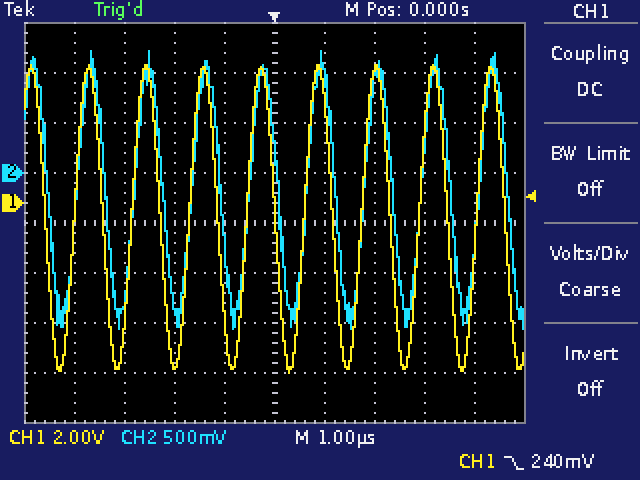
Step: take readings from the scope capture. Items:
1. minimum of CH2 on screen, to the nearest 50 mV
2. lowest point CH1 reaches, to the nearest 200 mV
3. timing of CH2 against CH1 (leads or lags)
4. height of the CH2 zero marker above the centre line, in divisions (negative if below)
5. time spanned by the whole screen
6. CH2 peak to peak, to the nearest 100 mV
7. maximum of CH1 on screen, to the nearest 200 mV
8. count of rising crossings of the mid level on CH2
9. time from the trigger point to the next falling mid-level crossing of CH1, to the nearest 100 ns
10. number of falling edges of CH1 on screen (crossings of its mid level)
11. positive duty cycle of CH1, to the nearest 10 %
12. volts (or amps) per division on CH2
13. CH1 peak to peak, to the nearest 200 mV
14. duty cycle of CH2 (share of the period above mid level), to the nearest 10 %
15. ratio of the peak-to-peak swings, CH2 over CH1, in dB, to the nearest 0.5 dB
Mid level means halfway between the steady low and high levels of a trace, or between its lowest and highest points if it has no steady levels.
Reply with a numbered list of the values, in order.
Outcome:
1. -1.55 V
2. -6.8 V
3. lags
4. +1.0 div
5. 10 µs
6. 2.80 V
7. 5.6 V
8. 8
9. 1.2 µs
10. 9
11. 50 %
12. 500 mV
13. 12.4 V
14. 50 %
15. -13.0 dB
